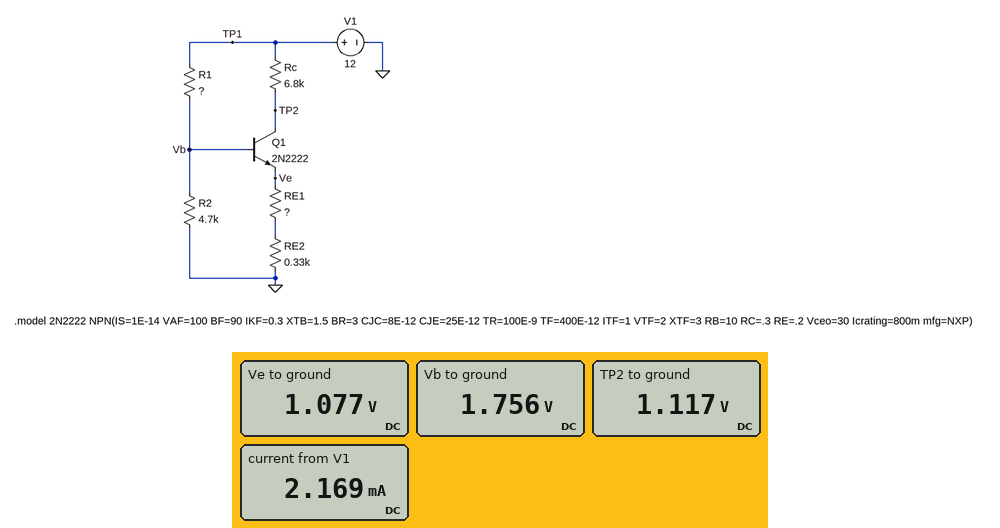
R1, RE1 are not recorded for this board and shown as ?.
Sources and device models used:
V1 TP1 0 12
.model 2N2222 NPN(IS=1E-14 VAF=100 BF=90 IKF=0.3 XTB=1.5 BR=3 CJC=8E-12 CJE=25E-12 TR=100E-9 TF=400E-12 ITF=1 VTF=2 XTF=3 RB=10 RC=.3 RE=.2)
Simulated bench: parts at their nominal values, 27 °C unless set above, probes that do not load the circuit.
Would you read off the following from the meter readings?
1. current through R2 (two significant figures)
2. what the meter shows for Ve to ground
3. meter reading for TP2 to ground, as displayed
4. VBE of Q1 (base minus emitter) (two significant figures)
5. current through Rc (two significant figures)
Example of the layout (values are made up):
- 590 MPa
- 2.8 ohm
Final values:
- 370 µA
- 1.077 V
- 1.117 V
- 680 mV
- 1.6 mA
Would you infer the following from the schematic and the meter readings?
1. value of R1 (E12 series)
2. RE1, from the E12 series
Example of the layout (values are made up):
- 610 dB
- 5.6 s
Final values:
- 18 kΩ
- 270 Ω
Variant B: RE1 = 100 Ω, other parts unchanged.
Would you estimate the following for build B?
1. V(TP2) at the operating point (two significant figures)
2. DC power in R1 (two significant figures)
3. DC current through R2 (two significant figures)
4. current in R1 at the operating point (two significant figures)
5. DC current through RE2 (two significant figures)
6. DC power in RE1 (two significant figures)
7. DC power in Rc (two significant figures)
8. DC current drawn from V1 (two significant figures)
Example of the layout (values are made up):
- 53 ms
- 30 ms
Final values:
- 850 mV
- 6.1 mW
- 320 µA
- 580 µA
- 1.9 mA
- 360 µW
- 18 mW
- 2.2 mA
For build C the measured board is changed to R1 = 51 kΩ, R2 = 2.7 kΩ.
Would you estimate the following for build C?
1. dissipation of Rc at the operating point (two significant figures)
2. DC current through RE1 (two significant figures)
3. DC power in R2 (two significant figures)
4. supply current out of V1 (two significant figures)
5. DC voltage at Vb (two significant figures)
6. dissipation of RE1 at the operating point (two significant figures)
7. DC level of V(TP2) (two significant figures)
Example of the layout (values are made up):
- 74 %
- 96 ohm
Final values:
- 15 µW
- 48 µA
- 130 µW
- 270 µA
- 600 mV
- 620 nW
- 12 V
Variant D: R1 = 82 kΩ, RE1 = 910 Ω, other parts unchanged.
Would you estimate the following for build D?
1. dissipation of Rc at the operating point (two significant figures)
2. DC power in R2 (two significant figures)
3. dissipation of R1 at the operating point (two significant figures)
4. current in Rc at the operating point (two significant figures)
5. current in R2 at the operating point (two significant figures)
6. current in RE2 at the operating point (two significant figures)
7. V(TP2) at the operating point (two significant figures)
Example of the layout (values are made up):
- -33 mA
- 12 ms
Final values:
- 21 µW
- 89 µW
- 1.6 mW
- 56 µA
- 140 µA
- 57 µA
- 12 V
